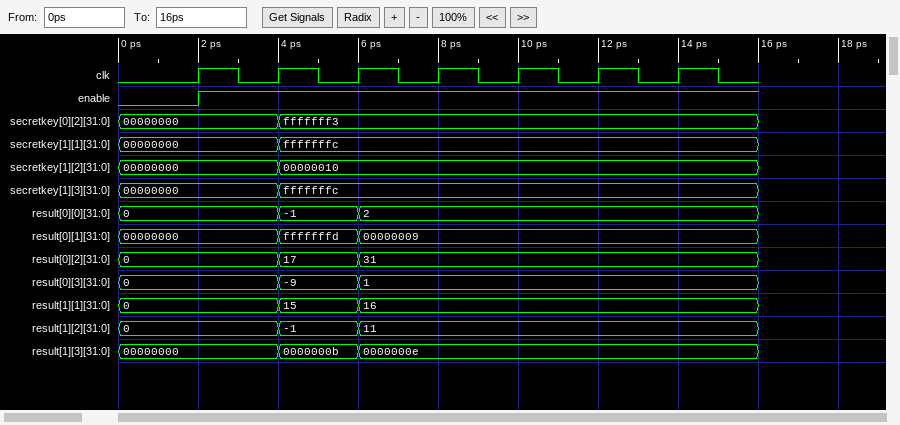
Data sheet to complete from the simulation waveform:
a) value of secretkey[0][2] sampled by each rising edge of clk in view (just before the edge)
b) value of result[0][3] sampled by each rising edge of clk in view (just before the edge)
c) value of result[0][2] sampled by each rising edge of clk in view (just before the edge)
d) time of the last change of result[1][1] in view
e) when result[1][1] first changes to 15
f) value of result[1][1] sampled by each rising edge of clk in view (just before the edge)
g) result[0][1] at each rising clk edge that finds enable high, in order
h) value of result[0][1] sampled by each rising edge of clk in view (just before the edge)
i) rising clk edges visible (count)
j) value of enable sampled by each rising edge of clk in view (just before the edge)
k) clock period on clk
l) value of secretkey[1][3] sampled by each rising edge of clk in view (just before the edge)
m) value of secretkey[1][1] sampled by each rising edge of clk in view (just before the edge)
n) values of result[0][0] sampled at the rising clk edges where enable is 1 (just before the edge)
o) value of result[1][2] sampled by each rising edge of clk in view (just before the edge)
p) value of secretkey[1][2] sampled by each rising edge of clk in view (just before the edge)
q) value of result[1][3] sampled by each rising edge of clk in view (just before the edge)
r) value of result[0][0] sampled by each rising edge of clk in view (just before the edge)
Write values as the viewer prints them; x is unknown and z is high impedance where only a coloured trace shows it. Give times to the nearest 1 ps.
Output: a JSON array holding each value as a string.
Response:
["00000000, 00000000, fffffff3, fffffff3, fffffff3, fffffff3, fffffff3", "0, 0, -9, 1, 1, 1, 1", "0, 0, 17, 31, 31, 31, 31", "6 ps", "4 ps", "0, 0, 15, 16, 16, 16, 16", "00000000, fffffffd, 00000009, 00000009, 00000009, 00000009", "00000000, 00000000, fffffffd, 00000009, 00000009, 00000009, 00000009", "7", "0 1 1 1 1 1 1", "2 ps", "00000000, 00000000, fffffffc, fffffffc, fffffffc, fffffffc, fffffffc", "00000000, 00000000, fffffffc, fffffffc, fffffffc, fffffffc, fffffffc", "0, -1, 2, 2, 2, 2", "0, 0, -1, 11, 11, 11, 11", "00000000, 00000000, 00000010, 00000010, 00000010, 00000010, 00000010", "00000000, 00000000, 0000000b, 0000000e, 0000000e, 0000000e, 0000000e", "0, 0, -1, 2, 2, 2, 2"]
